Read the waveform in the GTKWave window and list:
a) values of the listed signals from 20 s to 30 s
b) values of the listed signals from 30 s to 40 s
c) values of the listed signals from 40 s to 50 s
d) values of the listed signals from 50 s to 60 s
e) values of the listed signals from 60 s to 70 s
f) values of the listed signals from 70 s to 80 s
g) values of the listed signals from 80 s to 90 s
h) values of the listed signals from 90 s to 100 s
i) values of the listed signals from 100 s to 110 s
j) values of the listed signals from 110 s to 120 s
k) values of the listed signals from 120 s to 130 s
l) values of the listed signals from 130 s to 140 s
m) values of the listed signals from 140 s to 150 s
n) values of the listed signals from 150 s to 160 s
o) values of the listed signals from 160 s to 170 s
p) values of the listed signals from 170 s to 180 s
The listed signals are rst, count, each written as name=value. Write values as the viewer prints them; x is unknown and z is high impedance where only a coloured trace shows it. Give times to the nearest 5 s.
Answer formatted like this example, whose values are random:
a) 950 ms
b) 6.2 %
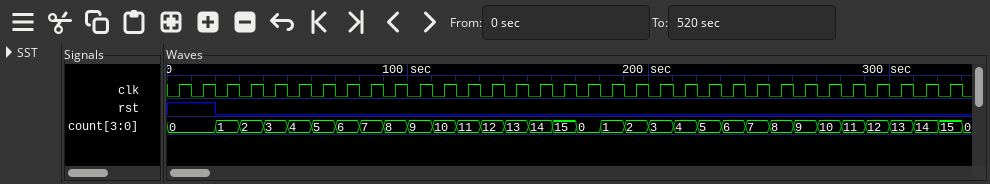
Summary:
a) rst=0, count=1
b) rst=0, count=2
c) rst=0, count=3
d) rst=0, count=4
e) rst=0, count=5
f) rst=0, count=6
g) rst=0, count=7
h) rst=0, count=8
i) rst=0, count=9
j) rst=0, count=10
k) rst=0, count=11
l) rst=0, count=12
m) rst=0, count=13
n) rst=0, count=14
o) rst=0, count=15
p) rst=0, count=0
